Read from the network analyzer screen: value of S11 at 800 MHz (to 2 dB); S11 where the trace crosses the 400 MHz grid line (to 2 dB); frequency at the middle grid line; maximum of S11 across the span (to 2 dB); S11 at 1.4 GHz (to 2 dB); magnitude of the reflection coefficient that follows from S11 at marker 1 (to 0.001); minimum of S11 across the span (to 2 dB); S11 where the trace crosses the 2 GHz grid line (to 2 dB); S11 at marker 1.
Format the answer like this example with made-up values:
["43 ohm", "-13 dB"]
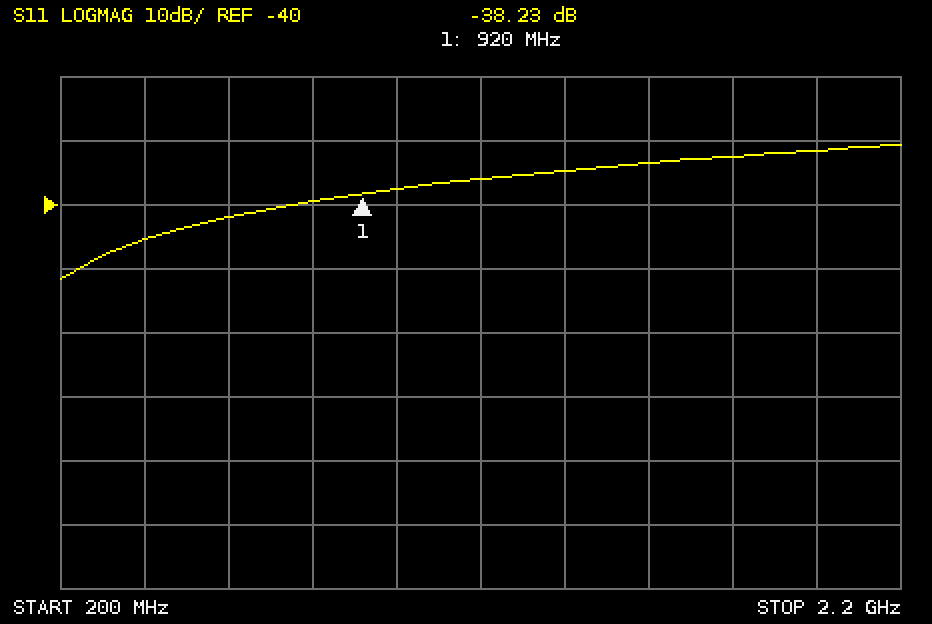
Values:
["-40 dB", "-46 dB", "1.2 GHz", "-30 dB", "-34 dB", "0.012", "-52 dB", "-32 dB", "-38.23 dB"]
